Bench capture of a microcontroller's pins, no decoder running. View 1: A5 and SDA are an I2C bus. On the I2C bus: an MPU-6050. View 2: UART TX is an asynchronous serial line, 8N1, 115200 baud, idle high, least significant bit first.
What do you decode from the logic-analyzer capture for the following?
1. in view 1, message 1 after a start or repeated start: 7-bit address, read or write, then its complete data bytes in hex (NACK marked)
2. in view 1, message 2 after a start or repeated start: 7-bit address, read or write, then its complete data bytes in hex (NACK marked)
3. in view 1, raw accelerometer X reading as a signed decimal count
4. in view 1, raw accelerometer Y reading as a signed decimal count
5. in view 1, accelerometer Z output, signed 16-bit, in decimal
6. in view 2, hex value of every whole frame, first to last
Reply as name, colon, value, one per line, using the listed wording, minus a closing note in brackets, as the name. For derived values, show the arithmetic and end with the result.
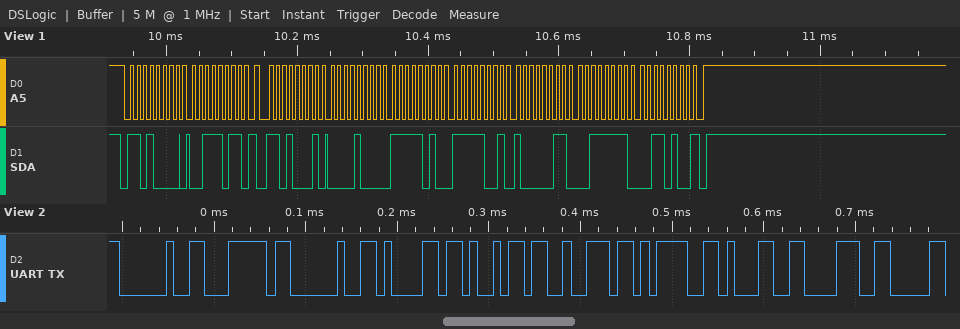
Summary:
in view 1, message 1 after a start or repeated start: 7-bit address, read or write, then its complete data bytes in hex: 0x68 write: 3B
in view 1, message 2 after a start or repeated start: 7-bit address, read or write, then its complete data bytes in hex: 0x68 read: 08 FA F9 83 3F 34 NACK
in view 1, raw accelerometer X reading as a signed decimal count: 0x08FA = 2298
in view 1, raw accelerometer Y reading as a signed decimal count: 0xF983 = -1661
in view 1, accelerometer Z output, signed 16-bit, in decimal: 0x3F34 = 16180
in view 2, hex value of every whole frame, first to last: 0x20 0x7C 0x20 0x61 0x69 0x72 0x3D 0x31 0x38
